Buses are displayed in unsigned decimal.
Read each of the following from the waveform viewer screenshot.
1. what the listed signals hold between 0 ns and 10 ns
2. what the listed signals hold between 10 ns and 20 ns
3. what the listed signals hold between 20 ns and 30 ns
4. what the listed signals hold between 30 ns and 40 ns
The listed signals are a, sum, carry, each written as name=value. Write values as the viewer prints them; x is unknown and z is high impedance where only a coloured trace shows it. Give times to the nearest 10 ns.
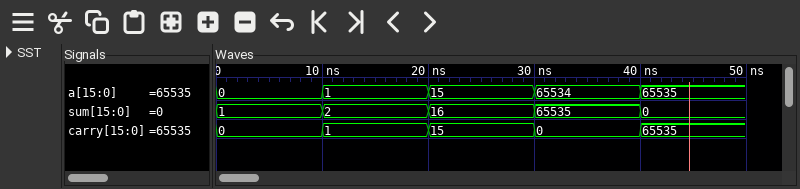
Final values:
a=0, sum=1, carry=0
a=1, sum=2, carry=1
a=15, sum=16, carry=15
a=65534, sum=65535, carry=0
